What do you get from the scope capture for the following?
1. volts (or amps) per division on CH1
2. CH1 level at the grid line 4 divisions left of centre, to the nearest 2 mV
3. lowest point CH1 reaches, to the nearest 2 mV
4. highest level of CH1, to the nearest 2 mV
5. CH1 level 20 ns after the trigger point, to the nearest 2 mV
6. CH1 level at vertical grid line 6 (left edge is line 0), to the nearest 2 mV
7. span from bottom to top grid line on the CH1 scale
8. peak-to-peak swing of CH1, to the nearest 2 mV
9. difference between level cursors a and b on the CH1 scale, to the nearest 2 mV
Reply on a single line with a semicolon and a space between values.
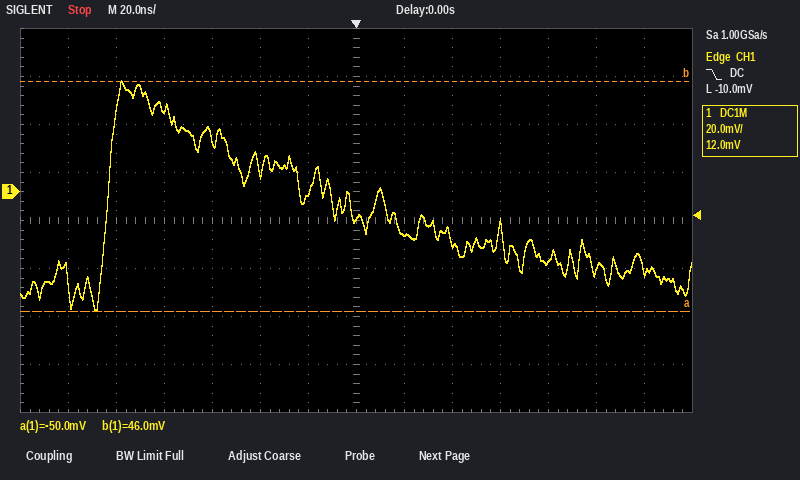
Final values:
20 mV; 34 mV; -50 mV; 46 mV; -18 mV; 0 mV; 160 mV; 96 mV; 96 mV
